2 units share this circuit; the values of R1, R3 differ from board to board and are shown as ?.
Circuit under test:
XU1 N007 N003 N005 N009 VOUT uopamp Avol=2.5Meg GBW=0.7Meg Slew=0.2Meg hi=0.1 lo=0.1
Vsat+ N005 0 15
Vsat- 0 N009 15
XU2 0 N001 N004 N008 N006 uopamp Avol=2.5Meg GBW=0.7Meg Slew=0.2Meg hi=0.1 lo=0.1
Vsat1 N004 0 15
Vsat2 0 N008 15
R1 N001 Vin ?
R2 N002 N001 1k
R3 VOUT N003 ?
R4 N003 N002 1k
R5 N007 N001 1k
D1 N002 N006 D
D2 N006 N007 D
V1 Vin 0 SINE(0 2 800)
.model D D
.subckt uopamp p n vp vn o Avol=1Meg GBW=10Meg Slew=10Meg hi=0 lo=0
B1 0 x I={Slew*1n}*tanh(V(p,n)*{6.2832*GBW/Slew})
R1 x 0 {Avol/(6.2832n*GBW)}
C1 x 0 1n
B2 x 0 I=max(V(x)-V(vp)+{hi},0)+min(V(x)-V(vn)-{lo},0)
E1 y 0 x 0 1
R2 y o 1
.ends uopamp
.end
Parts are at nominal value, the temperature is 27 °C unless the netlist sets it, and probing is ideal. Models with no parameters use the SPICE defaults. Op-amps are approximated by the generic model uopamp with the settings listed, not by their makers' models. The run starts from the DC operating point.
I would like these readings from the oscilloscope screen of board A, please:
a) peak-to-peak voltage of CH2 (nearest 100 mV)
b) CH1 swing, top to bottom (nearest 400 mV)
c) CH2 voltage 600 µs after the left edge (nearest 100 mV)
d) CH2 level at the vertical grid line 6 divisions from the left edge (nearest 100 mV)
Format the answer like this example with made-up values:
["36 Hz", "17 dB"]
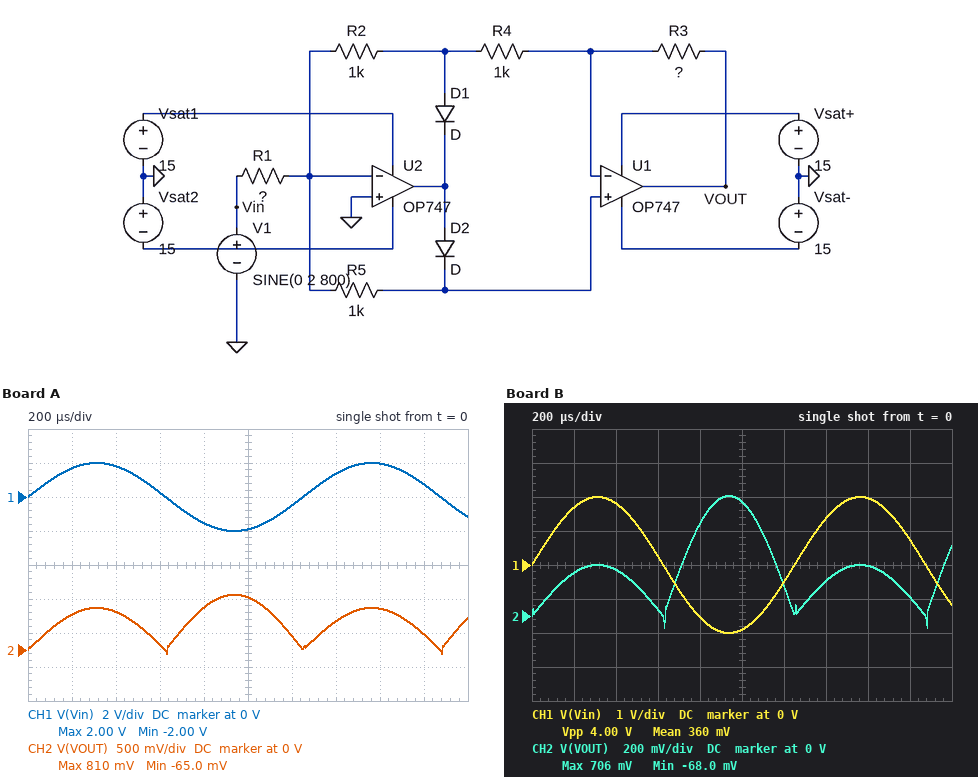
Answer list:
["900 mV", "4.0 V", "100 mV", "200 mV"]
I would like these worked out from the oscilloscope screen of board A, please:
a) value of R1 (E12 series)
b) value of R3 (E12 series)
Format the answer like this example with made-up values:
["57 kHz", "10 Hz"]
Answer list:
["2.2 kΩ", "680 Ω"]
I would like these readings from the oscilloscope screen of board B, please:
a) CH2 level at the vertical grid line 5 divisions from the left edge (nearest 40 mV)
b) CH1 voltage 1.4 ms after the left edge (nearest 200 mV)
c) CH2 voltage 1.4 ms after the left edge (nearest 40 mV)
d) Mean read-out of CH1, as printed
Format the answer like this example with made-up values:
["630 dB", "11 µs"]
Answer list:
["680 mV", "1.4 V", "200 mV", "360 mV"]
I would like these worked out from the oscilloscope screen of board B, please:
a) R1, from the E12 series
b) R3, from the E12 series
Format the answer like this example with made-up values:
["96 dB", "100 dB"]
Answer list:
["2.2 kΩ", "330 Ω"]
